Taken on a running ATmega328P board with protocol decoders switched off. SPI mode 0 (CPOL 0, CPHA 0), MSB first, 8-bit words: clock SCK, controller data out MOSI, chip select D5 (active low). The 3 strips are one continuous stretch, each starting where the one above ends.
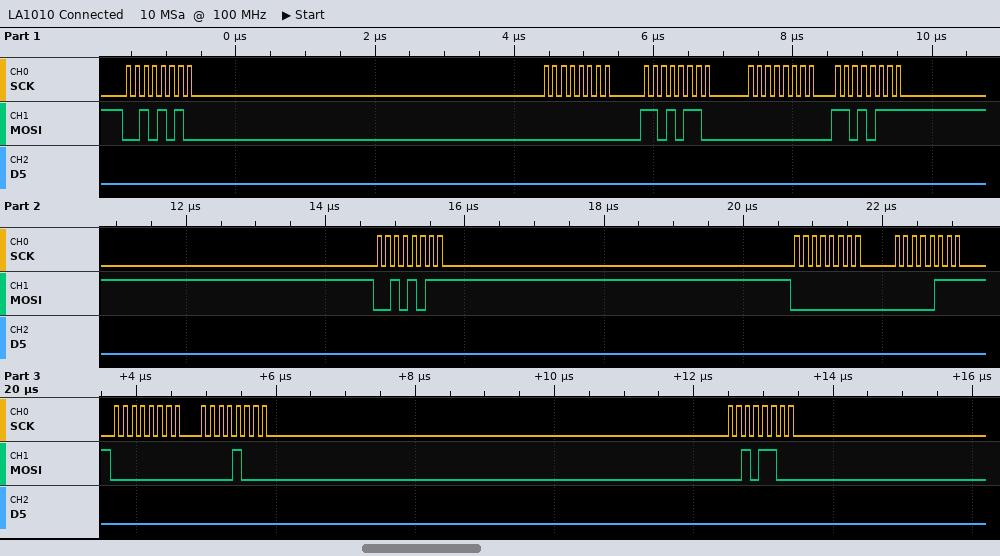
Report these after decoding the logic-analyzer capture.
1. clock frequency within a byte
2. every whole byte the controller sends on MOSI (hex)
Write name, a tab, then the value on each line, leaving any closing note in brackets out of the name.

clock frequency within a byte	8 MHz
every whole byte the controller sends on MOSI	2A 00 D6 00 D7 2B 00 07 00 08 2C
